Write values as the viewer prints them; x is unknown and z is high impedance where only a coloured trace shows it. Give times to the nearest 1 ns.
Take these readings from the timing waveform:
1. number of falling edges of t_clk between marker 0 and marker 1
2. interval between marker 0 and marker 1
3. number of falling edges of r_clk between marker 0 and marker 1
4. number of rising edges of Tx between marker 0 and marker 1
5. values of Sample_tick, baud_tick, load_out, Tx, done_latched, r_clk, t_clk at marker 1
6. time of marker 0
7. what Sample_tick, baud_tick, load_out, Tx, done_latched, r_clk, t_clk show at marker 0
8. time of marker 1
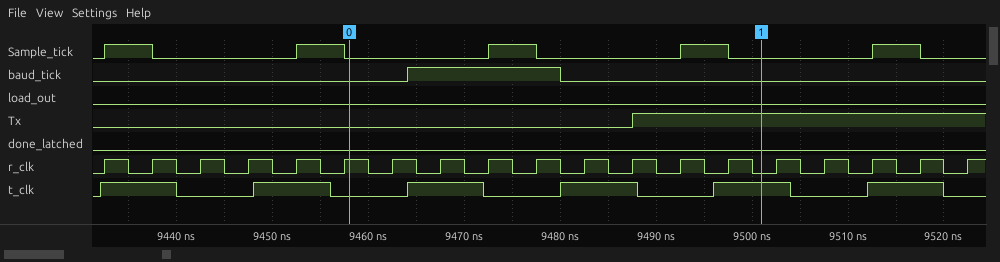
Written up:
2
43 ns
9
1
Sample_tick=0, baud_tick=0, load_out=0, Tx=1, done_latched=0, r_clk=0, t_clk=1
9458 ns
Sample_tick=0, baud_tick=0, load_out=0, Tx=0, done_latched=0, r_clk=1, t_clk=0
9501 ns
